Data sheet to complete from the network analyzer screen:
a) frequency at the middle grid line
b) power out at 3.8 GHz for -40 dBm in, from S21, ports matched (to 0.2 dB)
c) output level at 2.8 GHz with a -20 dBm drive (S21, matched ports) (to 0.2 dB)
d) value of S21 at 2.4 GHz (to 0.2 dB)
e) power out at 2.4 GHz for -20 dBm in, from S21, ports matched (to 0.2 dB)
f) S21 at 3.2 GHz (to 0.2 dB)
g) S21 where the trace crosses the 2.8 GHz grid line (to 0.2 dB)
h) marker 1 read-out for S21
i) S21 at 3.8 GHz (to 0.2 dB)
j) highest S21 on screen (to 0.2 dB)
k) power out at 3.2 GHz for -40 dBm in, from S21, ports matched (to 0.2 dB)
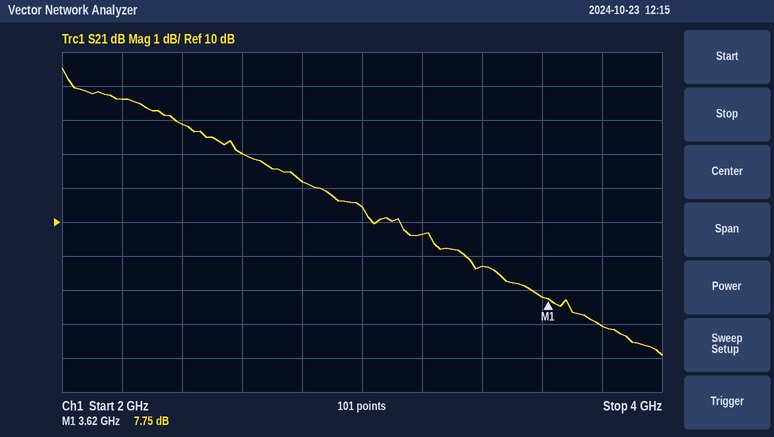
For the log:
3 GHz
-33.0 dBm
-8.8 dBm
12.8 dB
-7.2 dBm
9.6 dB
11.2 dB
7.75 dB
7.0 dB
14.6 dB
-30.4 dBm
